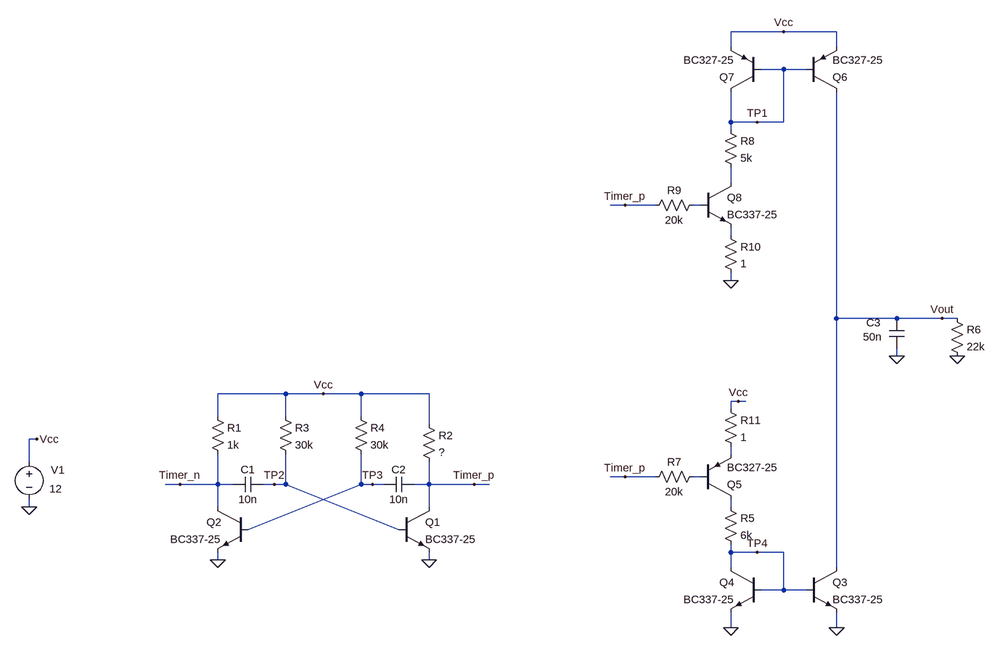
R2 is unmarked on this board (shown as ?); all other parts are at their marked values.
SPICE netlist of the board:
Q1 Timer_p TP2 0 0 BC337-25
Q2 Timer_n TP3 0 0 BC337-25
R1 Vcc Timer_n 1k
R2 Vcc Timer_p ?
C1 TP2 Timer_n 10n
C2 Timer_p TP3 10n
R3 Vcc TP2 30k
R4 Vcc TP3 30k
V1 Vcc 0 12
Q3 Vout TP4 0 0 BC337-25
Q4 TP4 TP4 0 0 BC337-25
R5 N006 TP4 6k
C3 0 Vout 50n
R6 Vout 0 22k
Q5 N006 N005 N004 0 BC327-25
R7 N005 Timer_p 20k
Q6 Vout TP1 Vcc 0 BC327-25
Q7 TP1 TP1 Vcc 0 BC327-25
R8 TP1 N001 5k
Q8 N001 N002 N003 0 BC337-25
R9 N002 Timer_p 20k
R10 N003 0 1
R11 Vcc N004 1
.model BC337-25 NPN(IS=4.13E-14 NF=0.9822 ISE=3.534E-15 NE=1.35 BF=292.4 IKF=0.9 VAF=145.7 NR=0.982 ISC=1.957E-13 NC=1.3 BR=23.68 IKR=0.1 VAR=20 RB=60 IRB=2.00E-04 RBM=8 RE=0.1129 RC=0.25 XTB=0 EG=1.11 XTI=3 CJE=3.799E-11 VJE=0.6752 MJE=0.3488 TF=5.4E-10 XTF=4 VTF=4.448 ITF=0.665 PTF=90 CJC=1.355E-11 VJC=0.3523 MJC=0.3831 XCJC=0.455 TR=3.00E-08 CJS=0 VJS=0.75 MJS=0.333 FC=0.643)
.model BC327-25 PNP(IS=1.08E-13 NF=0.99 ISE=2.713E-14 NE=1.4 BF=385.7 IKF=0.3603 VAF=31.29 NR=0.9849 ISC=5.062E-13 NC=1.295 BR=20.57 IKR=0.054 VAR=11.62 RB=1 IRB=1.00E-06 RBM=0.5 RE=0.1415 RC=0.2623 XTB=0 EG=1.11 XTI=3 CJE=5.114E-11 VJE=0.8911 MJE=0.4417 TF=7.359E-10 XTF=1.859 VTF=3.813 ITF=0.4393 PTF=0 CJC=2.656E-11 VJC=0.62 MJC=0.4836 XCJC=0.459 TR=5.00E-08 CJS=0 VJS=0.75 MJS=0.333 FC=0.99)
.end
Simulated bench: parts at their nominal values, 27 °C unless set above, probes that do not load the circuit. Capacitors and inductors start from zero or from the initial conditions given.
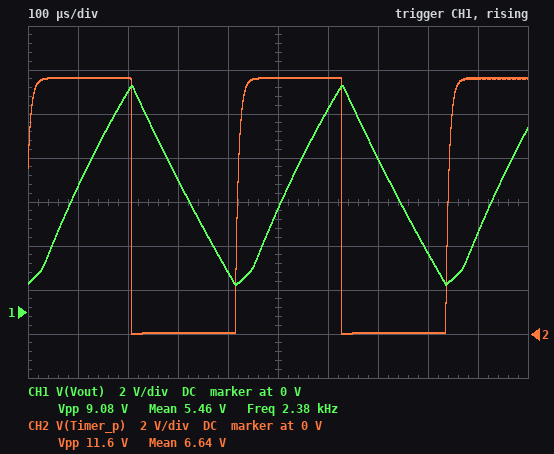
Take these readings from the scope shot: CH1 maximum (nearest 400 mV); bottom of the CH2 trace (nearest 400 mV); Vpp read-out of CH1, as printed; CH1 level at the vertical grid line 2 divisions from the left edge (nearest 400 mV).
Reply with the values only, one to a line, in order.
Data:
10.4 V
0 V
9.08 V
10.0 V
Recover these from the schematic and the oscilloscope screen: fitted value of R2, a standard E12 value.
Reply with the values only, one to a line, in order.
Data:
680 Ω
